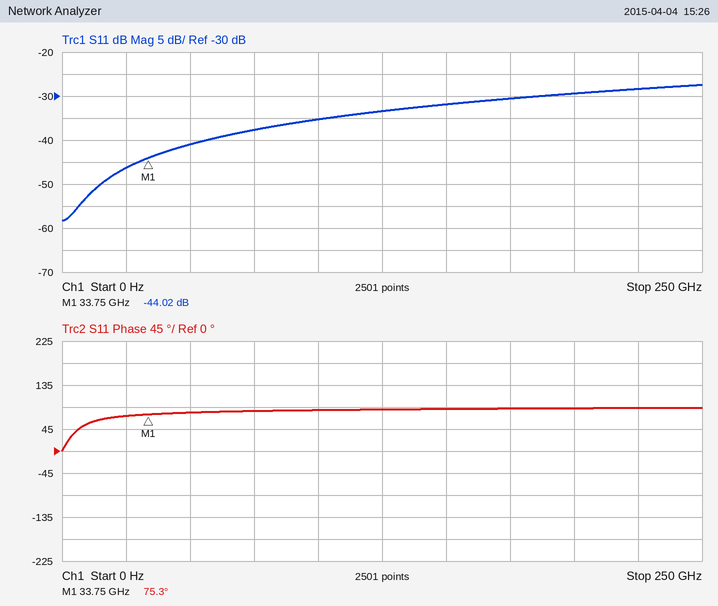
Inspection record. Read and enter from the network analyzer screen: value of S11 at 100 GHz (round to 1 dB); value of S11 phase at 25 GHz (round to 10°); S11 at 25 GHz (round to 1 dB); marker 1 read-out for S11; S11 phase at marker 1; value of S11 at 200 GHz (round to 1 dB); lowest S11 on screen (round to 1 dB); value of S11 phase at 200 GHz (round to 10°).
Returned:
-35 dB
70°
-46 dB
-44.02 dB
75.3°
-29 dB
-58 dB
90°
